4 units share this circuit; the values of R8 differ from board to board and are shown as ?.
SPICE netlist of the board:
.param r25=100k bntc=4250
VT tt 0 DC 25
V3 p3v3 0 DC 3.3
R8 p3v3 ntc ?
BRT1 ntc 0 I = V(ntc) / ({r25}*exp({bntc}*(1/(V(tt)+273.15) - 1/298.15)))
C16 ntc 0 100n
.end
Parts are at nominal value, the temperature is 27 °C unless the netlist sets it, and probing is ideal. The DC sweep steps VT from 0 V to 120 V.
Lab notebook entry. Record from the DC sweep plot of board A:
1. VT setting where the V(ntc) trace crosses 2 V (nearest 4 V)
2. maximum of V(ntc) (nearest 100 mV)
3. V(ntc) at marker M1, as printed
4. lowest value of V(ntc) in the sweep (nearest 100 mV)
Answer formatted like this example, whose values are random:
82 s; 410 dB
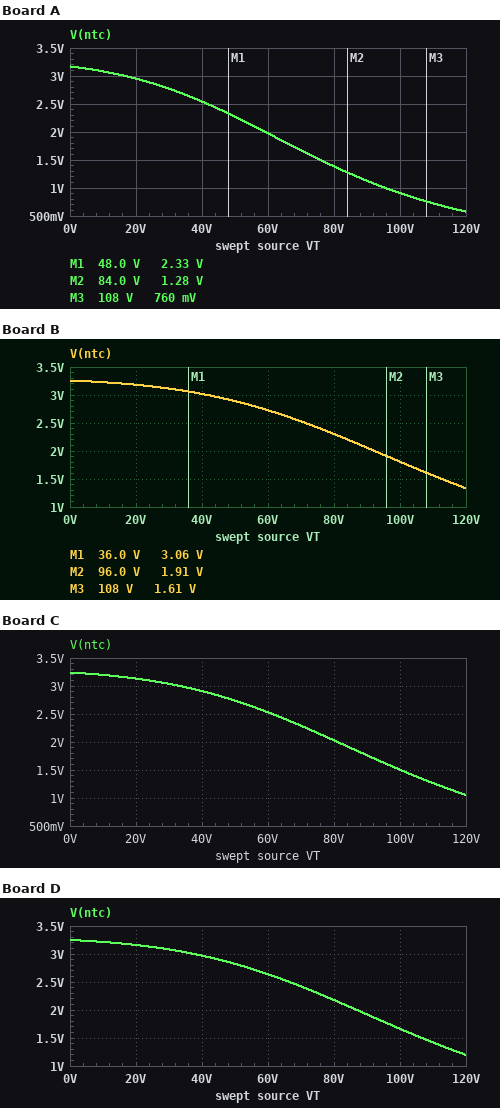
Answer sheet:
60 V; 3.2 V; 2.33 V; 600 mV
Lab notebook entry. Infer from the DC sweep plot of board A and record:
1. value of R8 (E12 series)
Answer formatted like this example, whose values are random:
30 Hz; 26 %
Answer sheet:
15 kΩ
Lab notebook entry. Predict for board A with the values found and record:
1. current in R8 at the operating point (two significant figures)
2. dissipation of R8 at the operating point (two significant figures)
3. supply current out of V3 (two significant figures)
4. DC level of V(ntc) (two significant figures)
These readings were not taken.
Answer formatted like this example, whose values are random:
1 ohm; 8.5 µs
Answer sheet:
29 µA; 12 µW; 29 µA; 2.9 V
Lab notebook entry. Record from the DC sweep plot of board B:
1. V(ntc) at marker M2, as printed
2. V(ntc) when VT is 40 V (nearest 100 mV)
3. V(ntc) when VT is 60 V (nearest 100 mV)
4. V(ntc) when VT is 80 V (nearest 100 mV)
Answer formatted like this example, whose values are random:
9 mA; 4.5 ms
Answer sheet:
1.91 V; 3.0 V; 2.7 V; 2.3 V
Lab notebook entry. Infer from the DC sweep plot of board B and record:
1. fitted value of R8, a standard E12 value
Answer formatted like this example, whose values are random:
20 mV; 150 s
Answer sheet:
4.7 kΩ
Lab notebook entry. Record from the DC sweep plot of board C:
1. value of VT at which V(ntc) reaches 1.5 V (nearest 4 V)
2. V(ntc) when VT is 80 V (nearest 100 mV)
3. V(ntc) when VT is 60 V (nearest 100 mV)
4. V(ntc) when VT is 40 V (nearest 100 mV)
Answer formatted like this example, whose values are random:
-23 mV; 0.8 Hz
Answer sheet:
100 V; 2.0 V; 2.5 V; 2.9 V
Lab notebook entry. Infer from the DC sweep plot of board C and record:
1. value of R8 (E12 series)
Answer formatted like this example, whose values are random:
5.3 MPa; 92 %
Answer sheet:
6.8 kΩ
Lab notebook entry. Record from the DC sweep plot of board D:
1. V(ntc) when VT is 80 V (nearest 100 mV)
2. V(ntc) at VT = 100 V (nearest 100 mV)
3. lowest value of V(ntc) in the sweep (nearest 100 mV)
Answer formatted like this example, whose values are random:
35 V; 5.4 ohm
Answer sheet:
2.2 V; 1.7 V; 1.2 V
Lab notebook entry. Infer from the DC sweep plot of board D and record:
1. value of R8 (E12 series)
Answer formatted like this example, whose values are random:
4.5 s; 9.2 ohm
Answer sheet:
5.6 kΩ
